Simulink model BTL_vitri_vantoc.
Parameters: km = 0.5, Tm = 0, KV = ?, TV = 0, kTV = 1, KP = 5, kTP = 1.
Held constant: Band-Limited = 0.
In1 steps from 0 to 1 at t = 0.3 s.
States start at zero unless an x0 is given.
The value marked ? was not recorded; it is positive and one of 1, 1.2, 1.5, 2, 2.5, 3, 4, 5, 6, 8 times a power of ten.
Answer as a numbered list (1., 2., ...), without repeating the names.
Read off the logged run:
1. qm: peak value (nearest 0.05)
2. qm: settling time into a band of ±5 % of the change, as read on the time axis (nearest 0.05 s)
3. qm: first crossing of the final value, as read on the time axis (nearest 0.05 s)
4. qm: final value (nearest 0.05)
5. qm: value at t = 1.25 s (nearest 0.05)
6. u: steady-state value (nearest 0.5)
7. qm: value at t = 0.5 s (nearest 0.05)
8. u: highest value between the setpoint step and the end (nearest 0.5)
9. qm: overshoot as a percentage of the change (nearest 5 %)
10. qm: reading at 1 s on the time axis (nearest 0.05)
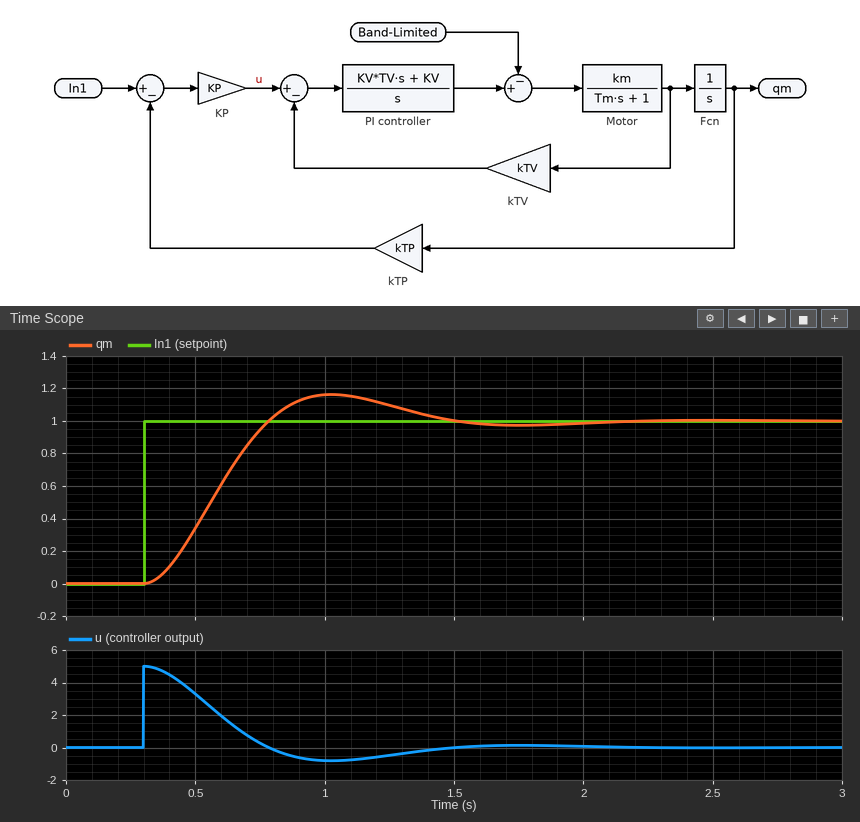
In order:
1. 1.15
2. 1.35 s
3. 0.80 s
4. 1.00
5. 1.10
6. 0.0
7. 0.35
8. 5.0
9. 15 %
10. 1.15
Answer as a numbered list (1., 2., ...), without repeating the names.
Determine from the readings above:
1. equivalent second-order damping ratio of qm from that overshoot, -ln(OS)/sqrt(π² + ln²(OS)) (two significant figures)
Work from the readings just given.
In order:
1. 0.52
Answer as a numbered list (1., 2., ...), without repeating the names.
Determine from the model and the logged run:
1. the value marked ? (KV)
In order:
1. 10
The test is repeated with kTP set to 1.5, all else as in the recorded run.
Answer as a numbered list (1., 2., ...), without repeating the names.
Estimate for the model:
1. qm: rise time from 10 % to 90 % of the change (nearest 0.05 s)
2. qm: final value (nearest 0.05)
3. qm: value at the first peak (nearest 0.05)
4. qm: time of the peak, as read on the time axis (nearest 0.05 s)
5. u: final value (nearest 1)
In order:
1. 0.25 s
2. 0.65
3. 0.85
4. 0.85 s
5. 0
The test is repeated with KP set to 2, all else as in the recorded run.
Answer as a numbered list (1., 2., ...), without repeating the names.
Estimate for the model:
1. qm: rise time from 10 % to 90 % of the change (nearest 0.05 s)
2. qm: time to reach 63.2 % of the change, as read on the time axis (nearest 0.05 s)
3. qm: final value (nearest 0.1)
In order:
1. 0.75 s
2. 0.90 s
3. 1.0
